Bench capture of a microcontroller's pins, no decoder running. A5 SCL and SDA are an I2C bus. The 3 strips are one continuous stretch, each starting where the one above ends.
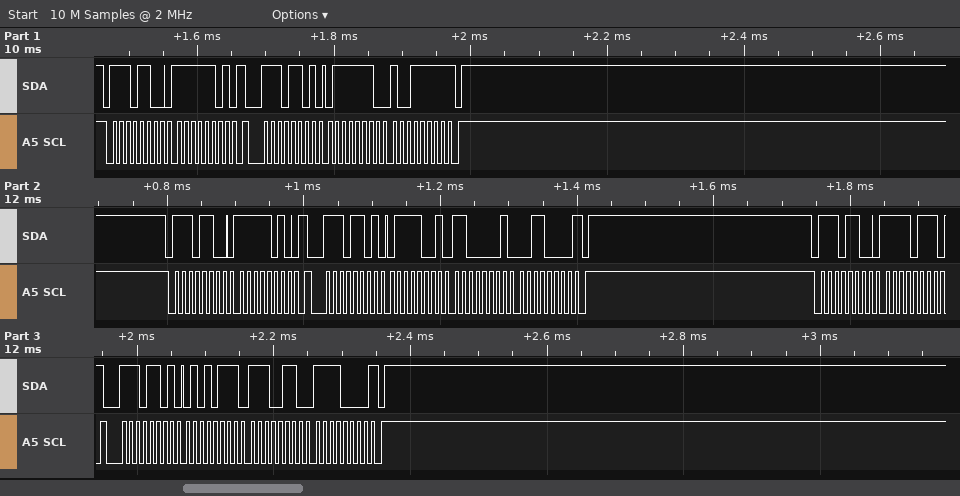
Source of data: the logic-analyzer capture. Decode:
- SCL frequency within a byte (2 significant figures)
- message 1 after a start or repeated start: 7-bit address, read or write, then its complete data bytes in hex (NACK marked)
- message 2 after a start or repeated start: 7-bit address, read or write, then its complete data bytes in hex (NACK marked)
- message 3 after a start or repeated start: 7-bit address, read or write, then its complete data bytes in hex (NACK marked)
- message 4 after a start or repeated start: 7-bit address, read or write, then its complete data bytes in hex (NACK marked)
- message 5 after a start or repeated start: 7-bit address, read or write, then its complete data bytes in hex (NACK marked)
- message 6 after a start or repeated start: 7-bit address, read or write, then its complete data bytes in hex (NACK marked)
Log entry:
100 kHz
0x76 write: FD
0x76 read: 7E 9F NACK
0x76 write: FA
0x76 read: 79 C1 30 NACK
0x76 write: F7
0x76 read: 57 E6 F0 NACK
